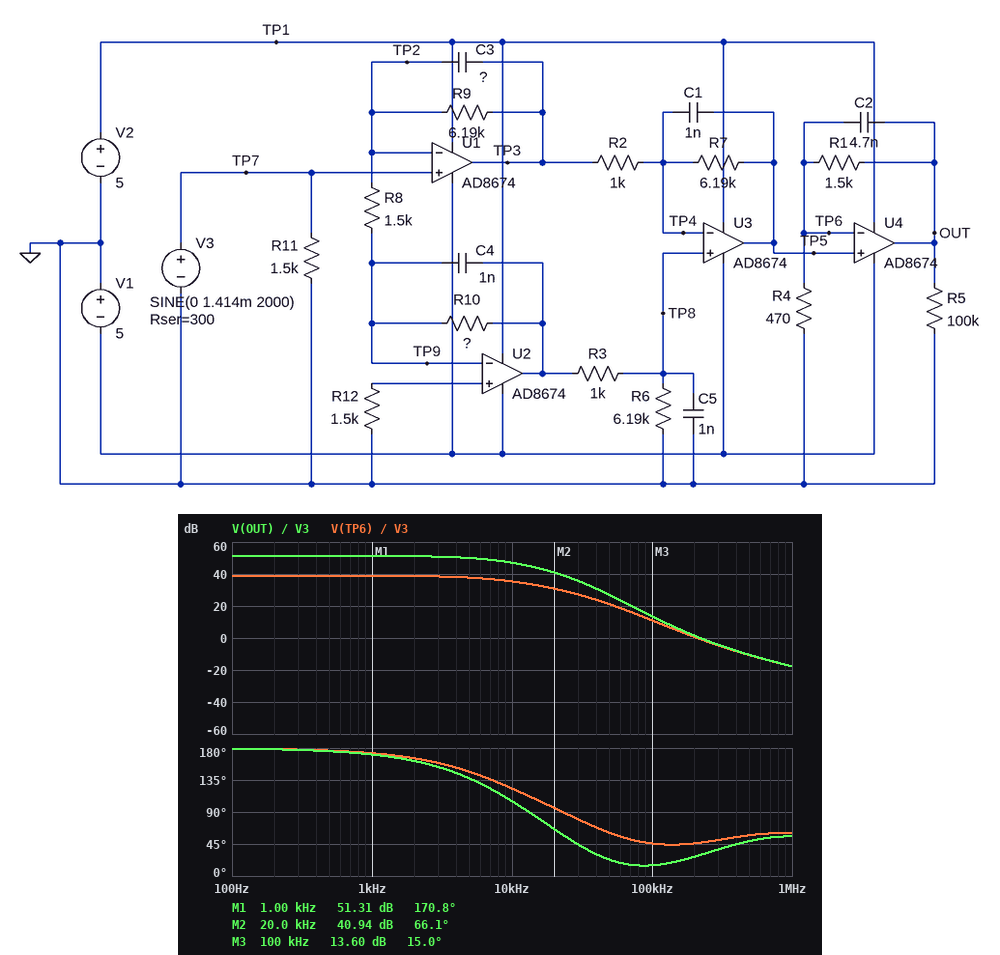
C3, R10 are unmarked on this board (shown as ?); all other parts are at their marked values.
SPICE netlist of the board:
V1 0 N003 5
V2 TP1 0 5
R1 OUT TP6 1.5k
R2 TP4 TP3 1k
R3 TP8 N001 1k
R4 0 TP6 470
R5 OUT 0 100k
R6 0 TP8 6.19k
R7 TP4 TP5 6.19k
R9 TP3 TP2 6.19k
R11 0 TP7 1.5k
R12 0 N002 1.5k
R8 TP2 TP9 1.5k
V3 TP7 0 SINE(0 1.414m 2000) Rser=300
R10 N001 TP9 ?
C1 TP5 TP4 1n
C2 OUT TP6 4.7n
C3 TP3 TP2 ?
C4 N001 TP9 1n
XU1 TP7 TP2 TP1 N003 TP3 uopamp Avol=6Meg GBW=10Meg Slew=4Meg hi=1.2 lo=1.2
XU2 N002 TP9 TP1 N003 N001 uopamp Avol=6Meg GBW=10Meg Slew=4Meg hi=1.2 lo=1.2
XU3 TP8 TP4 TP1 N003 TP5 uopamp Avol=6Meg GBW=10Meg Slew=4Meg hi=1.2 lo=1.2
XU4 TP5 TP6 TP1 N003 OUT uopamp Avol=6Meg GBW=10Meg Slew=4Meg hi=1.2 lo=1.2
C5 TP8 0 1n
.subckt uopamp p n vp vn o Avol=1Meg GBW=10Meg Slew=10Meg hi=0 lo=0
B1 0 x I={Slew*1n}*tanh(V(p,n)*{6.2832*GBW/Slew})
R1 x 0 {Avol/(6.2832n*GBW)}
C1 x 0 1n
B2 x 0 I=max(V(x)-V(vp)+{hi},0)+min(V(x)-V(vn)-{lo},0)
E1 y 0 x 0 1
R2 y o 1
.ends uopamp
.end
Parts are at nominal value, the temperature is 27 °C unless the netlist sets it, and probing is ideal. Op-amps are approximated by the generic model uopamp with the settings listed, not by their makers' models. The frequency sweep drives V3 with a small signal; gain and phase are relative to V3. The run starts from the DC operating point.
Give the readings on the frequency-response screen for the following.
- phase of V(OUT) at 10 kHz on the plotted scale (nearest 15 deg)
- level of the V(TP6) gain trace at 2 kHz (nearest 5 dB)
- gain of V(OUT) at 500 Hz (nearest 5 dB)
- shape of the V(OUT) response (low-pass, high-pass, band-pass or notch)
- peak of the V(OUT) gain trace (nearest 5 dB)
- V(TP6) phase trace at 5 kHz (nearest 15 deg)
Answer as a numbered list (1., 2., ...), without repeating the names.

1. 105 deg
2. 40 dB
3. 50 dB
4. low-pass
5. 50 dB
6. 150 deg
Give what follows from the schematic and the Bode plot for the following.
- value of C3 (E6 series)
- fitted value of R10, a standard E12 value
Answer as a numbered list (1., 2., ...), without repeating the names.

1. 680 pF
2. 18 kΩ
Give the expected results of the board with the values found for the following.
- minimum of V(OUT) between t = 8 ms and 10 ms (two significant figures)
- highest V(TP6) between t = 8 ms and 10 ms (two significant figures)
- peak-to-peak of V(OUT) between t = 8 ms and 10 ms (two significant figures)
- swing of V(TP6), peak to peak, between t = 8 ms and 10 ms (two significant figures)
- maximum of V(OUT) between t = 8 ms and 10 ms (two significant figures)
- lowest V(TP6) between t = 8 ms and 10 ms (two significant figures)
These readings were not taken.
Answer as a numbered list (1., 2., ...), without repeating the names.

1. -510 mV
2. 120 mV
3. 1.0 V
4. 240 mV
5. 510 mV
6. -120 mV
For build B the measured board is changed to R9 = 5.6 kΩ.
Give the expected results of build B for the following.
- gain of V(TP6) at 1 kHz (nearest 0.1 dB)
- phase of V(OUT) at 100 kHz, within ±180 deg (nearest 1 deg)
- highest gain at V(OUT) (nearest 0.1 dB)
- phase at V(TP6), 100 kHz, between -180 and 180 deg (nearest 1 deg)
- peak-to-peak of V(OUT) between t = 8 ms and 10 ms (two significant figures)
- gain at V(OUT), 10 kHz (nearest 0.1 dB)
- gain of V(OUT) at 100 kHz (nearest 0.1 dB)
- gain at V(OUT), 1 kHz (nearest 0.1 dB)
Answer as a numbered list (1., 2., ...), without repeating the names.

1. 38.7 dB
2. 16 deg
3. 51.2 dB
4. 47 deg
5. 990 mV
6. 46.8 dB
7. 13.6 dB
8. 51.1 dB
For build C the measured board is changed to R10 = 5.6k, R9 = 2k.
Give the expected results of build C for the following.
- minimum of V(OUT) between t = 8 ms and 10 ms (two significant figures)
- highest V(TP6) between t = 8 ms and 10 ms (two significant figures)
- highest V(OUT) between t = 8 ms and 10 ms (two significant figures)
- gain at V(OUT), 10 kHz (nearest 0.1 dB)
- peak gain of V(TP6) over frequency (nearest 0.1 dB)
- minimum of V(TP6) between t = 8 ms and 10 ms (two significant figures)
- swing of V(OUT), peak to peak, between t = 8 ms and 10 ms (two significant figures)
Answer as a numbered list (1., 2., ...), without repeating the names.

1. -180 mV
2. 44 mV
3. 180 mV
4. 40.6 dB
5. 29.9 dB
6. -44 mV
7. 370 mV
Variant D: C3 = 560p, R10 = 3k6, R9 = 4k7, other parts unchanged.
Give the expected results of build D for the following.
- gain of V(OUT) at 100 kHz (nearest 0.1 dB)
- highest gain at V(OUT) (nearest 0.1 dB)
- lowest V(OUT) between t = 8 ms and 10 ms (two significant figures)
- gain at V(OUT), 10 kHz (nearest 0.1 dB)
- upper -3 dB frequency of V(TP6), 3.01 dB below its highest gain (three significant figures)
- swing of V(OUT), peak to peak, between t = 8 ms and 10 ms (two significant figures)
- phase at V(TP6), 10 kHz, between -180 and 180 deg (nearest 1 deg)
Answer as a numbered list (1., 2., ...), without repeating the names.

1. 14.4 dB
2. 43.0 dB
3. -200 mV
4. 41.5 dB
5. 21.1 kHz
6. 400 mV
7. 149 deg
